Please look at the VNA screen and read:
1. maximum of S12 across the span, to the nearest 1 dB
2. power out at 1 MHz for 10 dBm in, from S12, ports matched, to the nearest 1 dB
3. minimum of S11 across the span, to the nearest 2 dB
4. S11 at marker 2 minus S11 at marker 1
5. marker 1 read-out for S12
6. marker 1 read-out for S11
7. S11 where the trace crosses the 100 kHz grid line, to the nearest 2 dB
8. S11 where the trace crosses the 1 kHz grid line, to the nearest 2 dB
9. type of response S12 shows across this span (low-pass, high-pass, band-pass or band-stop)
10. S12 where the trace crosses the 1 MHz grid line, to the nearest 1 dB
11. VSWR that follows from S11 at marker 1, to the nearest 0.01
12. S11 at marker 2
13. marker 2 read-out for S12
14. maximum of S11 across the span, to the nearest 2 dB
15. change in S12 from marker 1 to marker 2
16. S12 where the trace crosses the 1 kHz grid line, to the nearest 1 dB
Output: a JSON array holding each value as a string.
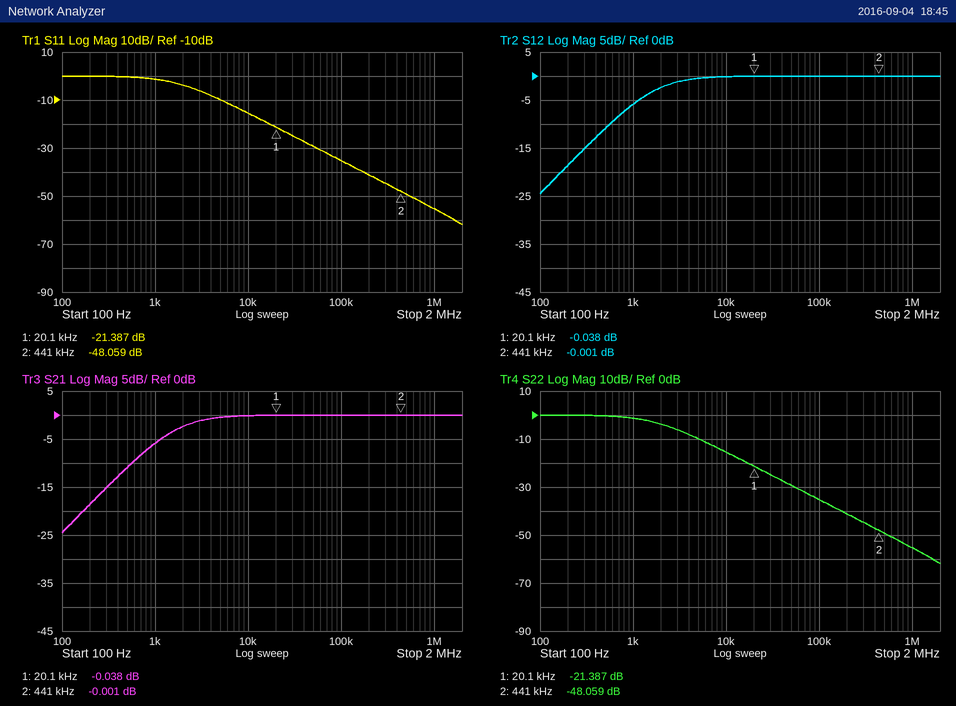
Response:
["0 dB", "10 dBm", "-62 dB", "-26.672 dB", "-0.038 dB", "-21.387 dB", "-36 dB", "-2 dB", "high-pass", "0 dB", "1.19", "-48.059 dB", "-0.001 dB", "0 dB", "0.037 dB", "-6 dB"]
